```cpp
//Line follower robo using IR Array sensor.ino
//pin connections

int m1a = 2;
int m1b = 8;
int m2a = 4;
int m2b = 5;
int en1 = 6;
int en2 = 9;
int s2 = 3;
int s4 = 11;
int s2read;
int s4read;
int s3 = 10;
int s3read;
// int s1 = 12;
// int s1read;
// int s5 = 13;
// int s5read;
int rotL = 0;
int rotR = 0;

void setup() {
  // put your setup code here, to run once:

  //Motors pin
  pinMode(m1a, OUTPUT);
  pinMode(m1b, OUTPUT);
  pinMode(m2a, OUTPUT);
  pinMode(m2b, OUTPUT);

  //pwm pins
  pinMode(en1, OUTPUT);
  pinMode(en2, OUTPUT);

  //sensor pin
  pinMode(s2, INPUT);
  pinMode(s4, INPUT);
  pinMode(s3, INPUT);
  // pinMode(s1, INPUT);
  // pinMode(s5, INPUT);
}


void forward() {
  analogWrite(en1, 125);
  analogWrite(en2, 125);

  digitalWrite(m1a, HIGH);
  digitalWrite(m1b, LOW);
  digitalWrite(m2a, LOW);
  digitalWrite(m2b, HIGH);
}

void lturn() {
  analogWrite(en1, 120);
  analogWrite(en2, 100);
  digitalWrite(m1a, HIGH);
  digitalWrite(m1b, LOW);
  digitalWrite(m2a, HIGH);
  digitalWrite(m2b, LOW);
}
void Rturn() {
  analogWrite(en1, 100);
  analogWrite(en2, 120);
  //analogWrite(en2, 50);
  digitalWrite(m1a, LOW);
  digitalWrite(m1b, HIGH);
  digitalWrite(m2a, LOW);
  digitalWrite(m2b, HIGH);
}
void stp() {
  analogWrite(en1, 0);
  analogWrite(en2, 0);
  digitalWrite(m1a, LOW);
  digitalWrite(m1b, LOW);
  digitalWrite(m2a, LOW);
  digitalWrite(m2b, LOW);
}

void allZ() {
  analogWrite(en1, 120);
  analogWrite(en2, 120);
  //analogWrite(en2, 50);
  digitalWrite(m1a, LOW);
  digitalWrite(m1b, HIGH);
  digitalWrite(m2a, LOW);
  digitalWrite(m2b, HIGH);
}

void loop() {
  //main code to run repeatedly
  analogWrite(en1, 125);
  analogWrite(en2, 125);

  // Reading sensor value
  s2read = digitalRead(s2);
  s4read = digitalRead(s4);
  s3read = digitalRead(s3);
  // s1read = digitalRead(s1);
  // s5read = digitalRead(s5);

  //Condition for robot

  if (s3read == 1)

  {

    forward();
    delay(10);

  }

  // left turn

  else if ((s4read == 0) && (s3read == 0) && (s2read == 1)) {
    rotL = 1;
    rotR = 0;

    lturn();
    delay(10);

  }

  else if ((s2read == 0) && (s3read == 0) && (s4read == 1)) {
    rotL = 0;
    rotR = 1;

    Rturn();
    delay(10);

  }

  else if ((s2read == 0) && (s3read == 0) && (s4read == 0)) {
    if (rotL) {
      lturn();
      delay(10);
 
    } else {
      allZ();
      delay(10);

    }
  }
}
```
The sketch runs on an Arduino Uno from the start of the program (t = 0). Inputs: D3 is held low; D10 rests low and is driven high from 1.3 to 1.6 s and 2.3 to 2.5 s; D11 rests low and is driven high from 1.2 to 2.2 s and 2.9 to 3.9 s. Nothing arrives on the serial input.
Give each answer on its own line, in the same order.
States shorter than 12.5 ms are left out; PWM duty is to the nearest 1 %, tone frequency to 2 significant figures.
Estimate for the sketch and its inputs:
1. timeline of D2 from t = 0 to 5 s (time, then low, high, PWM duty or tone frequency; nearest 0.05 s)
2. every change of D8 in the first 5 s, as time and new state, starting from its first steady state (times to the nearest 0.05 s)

0 s low; 1.3 s high; 1.6 s low; 2.3 s high; 2.5 s low
0 s high; 1.3 s low; 1.6 s high; 2.3 s low; 2.5 s high
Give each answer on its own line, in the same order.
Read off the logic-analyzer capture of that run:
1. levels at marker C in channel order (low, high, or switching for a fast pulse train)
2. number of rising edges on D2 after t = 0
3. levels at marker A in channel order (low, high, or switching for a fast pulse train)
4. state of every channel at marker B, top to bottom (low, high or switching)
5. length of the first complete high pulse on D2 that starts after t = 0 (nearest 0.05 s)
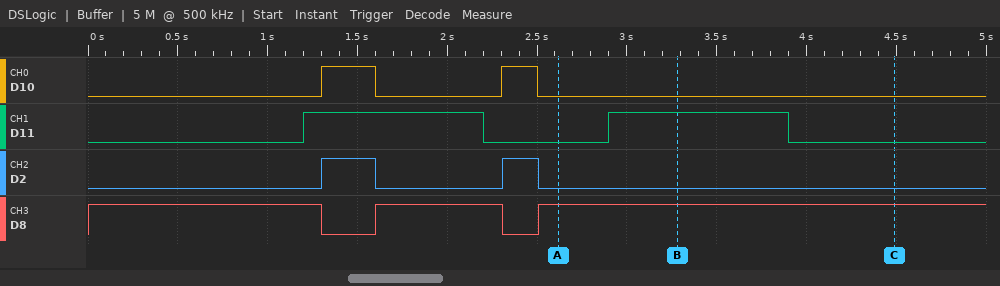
D10 low, D11 low, D2 low, D8 high
2
D10 low, D11 low, D2 low, D8 high
D10 low, D11 high, D2 low, D8 high
0.30 s
